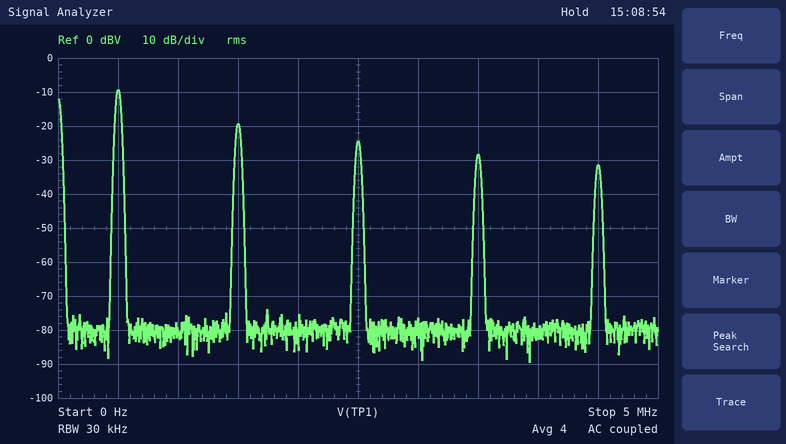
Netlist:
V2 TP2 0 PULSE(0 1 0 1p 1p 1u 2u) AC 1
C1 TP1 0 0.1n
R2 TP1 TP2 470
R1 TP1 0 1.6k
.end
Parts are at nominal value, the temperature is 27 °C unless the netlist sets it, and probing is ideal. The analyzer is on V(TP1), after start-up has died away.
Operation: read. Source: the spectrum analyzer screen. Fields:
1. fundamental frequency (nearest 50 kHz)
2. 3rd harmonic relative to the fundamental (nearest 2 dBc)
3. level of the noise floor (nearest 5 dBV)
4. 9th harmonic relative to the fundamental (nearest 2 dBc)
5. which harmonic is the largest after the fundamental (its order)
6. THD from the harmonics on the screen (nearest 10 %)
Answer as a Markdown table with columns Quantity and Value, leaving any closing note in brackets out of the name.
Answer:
| Quantity | Value |
|---|---|
| fundamental frequency | 500 kHz |
| 3rd harmonic relative to the fundamental | -10 dBc |
| level of the noise floor | -80 dBV |
| 9th harmonic relative to the fundamental | -22 dBc |
| which harmonic is the largest after the fundamental | 3 |
| THD from the harmonics on the screen | 40 % |
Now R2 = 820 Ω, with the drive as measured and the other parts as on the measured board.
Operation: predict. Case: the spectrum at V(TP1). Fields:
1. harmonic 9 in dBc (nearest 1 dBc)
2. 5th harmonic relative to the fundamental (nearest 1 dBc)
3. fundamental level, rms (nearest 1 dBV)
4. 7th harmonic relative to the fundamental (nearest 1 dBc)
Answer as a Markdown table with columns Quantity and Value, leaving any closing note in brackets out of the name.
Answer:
| Quantity | Value |
|---|---|
| harmonic 9 in dBc | -24 dBc |
| 5th harmonic relative to the fundamental | -16 dBc |
| fundamental level, rms | -11 dBV |
| 7th harmonic relative to the fundamental | -21 dBc |
